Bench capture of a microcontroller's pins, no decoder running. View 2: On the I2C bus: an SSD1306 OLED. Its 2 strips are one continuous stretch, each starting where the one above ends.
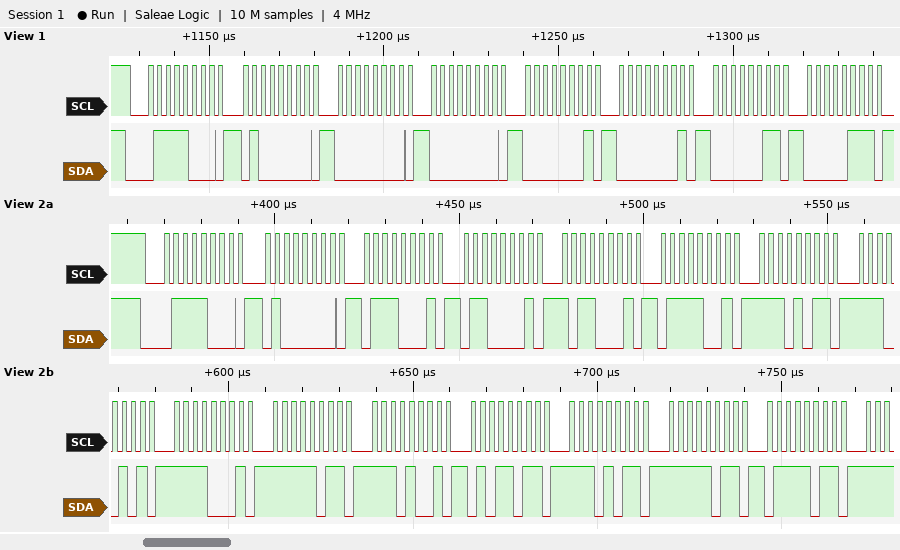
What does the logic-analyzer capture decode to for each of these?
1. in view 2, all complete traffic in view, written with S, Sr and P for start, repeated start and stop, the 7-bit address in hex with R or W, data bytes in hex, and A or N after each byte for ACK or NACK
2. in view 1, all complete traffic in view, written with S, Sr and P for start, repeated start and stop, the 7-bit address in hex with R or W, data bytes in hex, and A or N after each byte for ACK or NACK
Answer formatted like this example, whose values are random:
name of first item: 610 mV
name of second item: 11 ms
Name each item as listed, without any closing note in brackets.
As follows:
in view 2, all complete traffic in view, written with S, Sr and P for start, repeated start and stop, the 7-bit address in hex with R or W, data bytes in hex, and A or N after each byte for ACK or NACK: S 3CW A 40 A 71 A 61 A B1 A 79 A EB A E5 A F1 A FB A E9 A 5B A EB A FB A 7B A
in view 1, all complete traffic in view, written with S, Sr and P for start, repeated start and stop, the 7-bit address in hex with R or W, data bytes in hex, and A or N after each byte for ACK or NACK: S 3CW A 40 A 00 A 00 A 01 A 01 A 03 A 07 A
